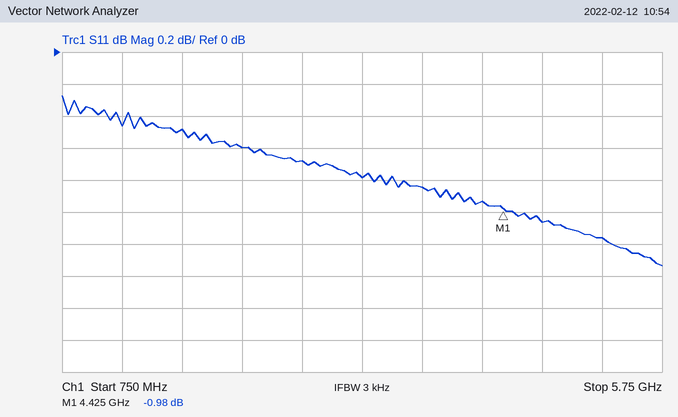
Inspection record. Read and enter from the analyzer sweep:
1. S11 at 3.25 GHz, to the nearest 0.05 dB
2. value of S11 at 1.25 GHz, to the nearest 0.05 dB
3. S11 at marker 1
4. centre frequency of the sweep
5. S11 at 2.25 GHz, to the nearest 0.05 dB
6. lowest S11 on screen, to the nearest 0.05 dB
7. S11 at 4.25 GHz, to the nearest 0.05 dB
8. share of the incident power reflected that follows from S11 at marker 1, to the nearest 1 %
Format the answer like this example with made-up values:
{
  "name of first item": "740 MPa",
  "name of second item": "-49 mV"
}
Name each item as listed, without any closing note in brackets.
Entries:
{
  "S11 at 3.25 GHz, to the nearest 0.05 dB": "-0.80 dB",
  "value of S11 at 1.25 GHz, to the nearest 0.05 dB": "-0.45 dB",
  "S11 at marker 1": "-0.98 dB",
  "centre frequency of the sweep": "3.25 GHz",
  "S11 at 2.25 GHz, to the nearest 0.05 dB": "-0.60 dB",
  "lowest S11 on screen, to the nearest 0.05 dB": "-1.35 dB",
  "S11 at 4.25 GHz, to the nearest 0.05 dB": "-0.95 dB",
  "share of the incident power reflected that follows from S11 at marker 1, to the nearest 1 %": "80 %"
}
